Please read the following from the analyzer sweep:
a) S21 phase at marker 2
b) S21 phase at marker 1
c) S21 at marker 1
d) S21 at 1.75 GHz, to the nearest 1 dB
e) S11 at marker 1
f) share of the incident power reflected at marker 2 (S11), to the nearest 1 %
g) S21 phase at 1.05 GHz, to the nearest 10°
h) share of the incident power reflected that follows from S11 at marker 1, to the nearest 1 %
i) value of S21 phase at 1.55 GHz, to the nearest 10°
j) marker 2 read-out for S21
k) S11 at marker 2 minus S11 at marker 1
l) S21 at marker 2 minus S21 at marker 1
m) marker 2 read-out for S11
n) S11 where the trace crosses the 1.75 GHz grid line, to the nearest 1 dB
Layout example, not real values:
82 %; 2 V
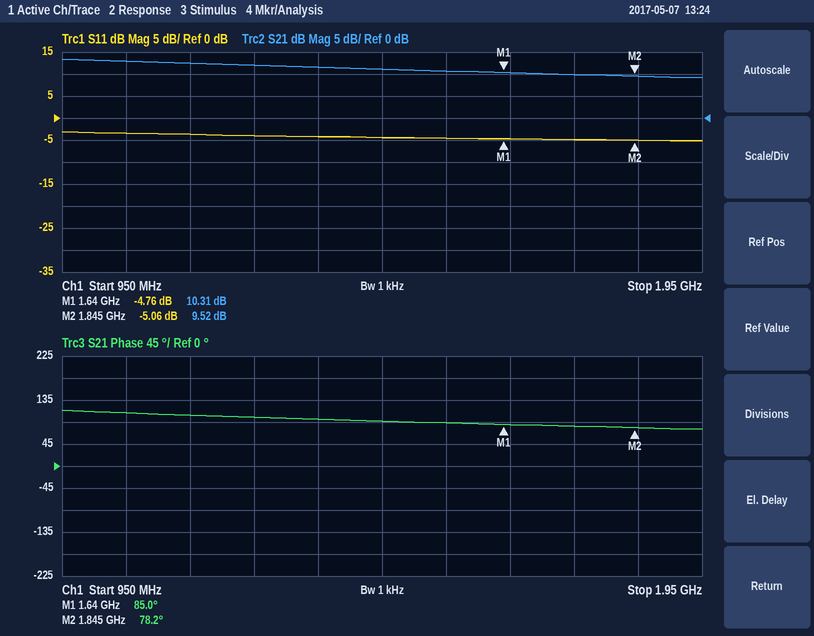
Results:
78.2°; 85.0°; 10.31 dB; 10 dB; -4.76 dB; 31 %; 110°; 33 %; 90°; 9.52 dB; -0.30 dB; -0.79 dB; -5.06 dB; -5 dB
